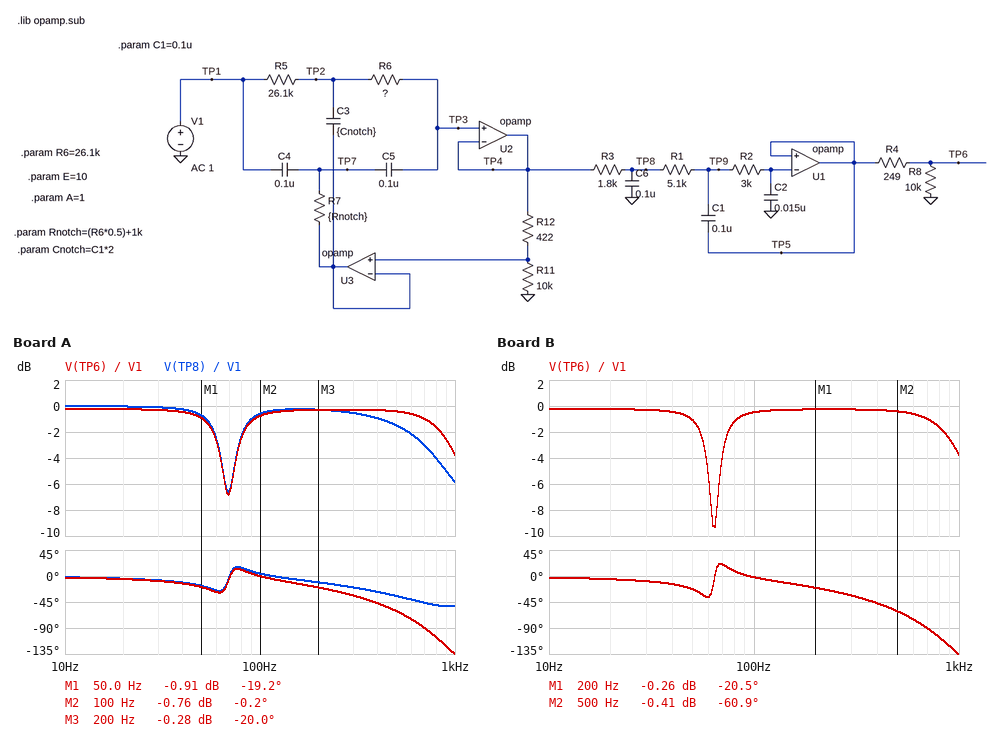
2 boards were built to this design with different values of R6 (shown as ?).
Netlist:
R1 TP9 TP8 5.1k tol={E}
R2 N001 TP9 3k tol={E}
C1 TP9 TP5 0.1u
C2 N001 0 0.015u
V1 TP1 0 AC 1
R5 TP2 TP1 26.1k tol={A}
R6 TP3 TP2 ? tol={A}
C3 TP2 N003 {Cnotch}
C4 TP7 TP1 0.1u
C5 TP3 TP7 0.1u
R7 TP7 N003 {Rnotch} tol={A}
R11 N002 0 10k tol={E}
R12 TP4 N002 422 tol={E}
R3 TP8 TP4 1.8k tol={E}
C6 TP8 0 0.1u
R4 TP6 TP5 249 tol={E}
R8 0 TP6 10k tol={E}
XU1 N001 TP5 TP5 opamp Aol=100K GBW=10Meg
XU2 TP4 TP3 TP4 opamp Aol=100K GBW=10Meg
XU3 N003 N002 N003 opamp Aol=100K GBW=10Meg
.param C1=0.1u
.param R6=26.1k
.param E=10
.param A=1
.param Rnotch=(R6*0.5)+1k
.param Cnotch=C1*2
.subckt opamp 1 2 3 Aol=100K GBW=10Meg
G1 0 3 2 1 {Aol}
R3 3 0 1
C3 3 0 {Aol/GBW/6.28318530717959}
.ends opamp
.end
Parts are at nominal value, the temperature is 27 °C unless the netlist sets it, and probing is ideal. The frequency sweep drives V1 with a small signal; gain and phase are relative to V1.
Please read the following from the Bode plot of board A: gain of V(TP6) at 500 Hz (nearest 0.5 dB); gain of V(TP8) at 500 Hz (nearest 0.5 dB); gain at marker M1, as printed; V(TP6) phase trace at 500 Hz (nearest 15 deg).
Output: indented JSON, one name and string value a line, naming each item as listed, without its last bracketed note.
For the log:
{
  "gain of V(TP6) at 500 Hz": "-0.5 dB",
  "gain of V(TP8) at 500 Hz": "-1.5 dB",
  "gain at marker M1, as printed": "-0.91 dB",
  "V(TP6) phase trace at 500 Hz": "-60 deg"
}
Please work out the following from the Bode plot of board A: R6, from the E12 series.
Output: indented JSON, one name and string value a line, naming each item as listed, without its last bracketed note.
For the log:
{
  "R6, from the E12 series": "18 kΩ"
}
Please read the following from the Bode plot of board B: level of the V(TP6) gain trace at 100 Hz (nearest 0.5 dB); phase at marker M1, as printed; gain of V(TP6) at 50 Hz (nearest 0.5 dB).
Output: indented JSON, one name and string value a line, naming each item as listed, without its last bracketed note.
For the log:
{
  "level of the V(TP6) gain trace at 100 Hz": "-0.5 dB",
  "phase at marker M1, as printed": "-20.5 deg",
  "gain of V(TP6) at 50 Hz": "-1.0 dB"
}
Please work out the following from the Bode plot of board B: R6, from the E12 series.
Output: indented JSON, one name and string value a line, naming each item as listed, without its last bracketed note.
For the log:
{
  "R6, from the E12 series": "22 kΩ"
}
